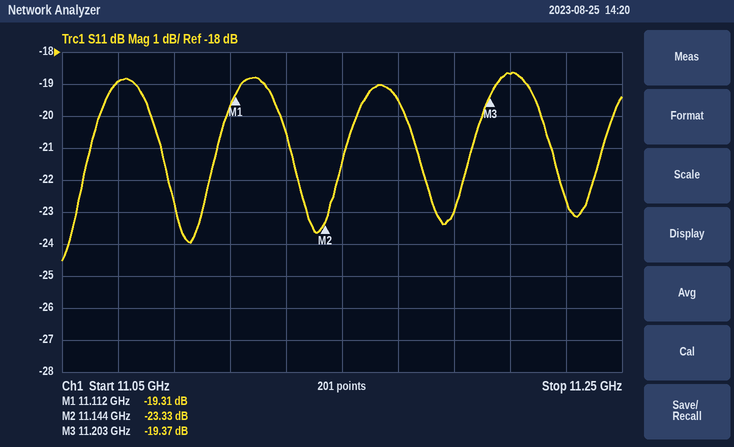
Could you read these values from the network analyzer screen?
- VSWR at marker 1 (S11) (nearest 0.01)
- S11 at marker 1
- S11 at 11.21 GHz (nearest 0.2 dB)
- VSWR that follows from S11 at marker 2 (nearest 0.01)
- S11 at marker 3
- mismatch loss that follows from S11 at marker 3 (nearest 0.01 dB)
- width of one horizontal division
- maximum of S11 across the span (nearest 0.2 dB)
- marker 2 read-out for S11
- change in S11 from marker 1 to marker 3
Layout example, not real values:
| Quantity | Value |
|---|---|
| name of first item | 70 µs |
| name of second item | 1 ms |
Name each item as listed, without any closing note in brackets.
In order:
| Quantity | Value |
|---|---|
| VSWR at marker 1 (S11) | 1.24 |
| S11 at marker 1 | -19.31 dB |
| S11 at 11.21 GHz | -18.6 dB |
| VSWR that follows from S11 at marker 2 | 1.15 |
| S11 at marker 3 | -19.37 dB |
| mismatch loss that follows from S11 at marker 3 | 0.05 dB |
| width of one horizontal division | 20 MHz |
| maximum of S11 across the span | -18.6 dB |
| marker 2 read-out for S11 | -23.33 dB |
| change in S11 from marker 1 to marker 3 | -0.06 dB |
